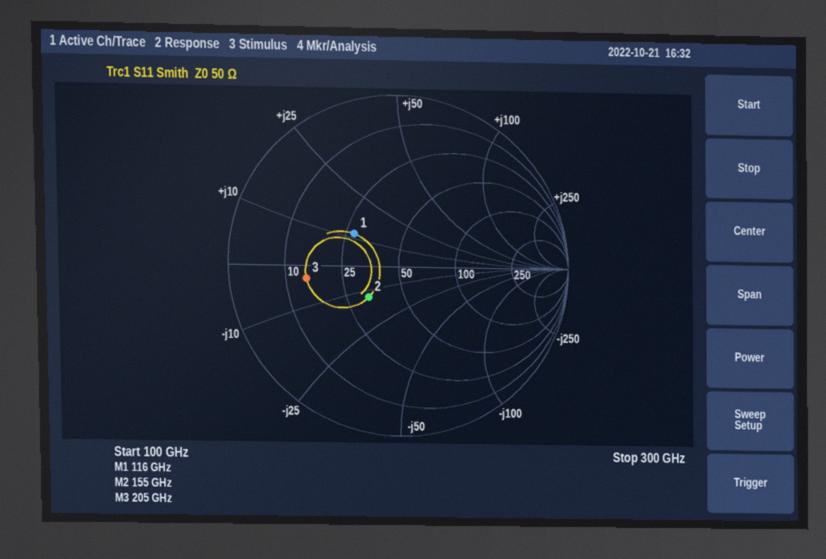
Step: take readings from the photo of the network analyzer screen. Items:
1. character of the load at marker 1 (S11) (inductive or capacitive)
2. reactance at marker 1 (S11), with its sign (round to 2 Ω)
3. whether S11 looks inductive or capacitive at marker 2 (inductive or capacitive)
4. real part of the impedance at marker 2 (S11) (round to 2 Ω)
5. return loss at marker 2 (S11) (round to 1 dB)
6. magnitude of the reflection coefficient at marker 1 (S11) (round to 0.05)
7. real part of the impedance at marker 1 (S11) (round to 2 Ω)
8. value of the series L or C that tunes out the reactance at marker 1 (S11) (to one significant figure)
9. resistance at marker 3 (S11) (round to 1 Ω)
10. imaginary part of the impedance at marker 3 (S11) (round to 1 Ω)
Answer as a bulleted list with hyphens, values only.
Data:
- inductive
- +12 Ω
- capacitive
- 32 Ω
- 12 dB
- 0.30
- 28 Ω
- 100 fF
- 15 Ω
- -3 Ω
